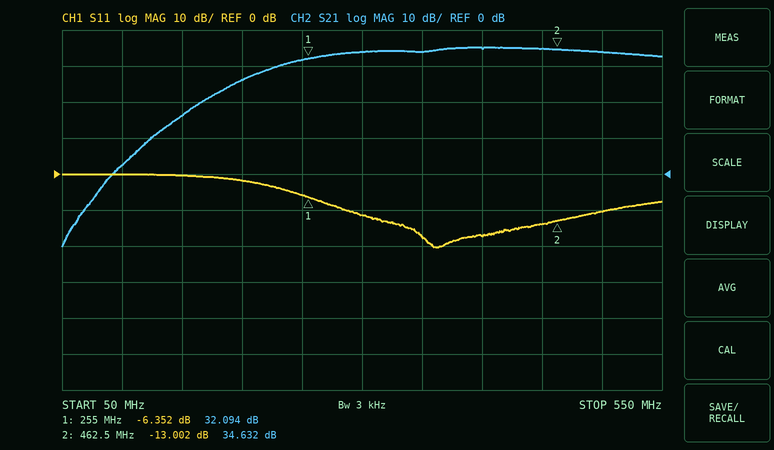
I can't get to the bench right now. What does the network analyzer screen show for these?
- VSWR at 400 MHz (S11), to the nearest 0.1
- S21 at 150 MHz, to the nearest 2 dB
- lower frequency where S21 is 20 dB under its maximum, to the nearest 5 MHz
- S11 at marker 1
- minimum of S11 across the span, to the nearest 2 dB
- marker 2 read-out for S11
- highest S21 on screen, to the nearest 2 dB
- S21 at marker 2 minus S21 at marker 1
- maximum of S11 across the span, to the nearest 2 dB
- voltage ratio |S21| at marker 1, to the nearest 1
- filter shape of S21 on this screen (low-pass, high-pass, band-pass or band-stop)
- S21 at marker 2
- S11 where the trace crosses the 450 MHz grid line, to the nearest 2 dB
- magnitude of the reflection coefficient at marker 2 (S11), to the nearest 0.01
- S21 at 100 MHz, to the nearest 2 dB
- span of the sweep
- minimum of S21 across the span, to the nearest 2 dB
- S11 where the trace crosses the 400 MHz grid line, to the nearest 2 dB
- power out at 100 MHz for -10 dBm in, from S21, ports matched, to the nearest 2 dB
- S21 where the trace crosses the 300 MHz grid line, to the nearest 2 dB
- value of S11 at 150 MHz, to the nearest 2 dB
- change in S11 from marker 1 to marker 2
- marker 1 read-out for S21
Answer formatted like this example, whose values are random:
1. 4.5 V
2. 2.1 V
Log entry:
1. 1.3
2. 16 dB
3. 145 MHz
4. -6.352 dB
5. -20 dB
6. -13.002 dB
7. 36 dB
8. 2.538 dB
9. 0 dB
10. 40
11. high-pass
12. 34.632 dB
13. -14 dB
14. 0.22
15. 2 dB
16. 500 MHz
17. -20 dB
18. -18 dB
19. -8 dBm
20. 34 dB
21. 0 dB
22. -6.650 dB
23. 32.094 dB
